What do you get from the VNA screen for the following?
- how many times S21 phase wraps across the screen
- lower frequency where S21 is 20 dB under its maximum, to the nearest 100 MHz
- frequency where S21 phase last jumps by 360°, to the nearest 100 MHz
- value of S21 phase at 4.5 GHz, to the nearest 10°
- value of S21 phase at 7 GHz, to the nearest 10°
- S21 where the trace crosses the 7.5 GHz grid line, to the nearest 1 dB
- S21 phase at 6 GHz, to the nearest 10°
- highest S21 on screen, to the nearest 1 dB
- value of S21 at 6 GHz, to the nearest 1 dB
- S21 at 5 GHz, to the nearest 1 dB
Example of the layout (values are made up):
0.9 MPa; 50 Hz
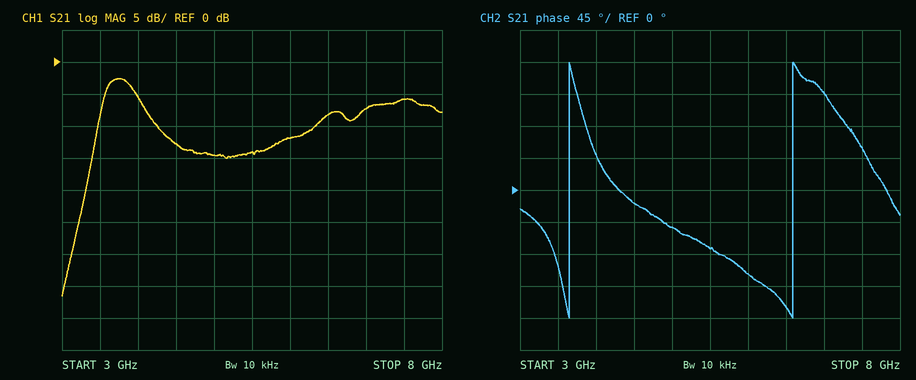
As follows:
2; 3.3 GHz; 6.6 GHz; -20°; 140°; -6 dB; -120°; -3 dB; -12 dB; -15 dB
